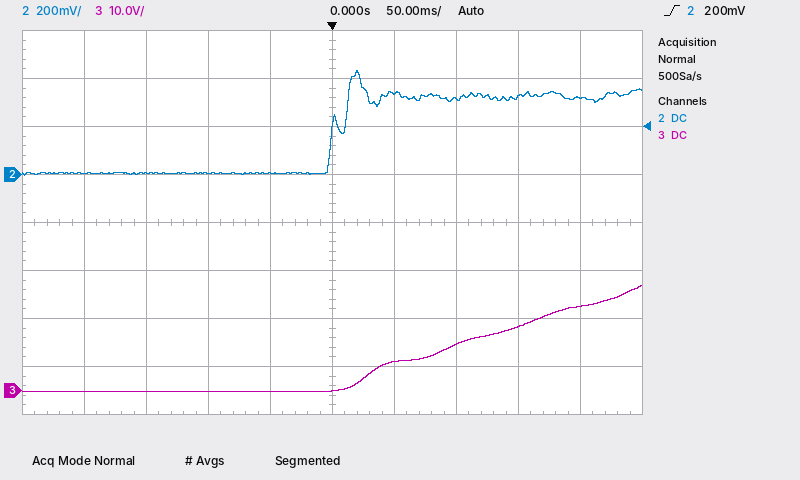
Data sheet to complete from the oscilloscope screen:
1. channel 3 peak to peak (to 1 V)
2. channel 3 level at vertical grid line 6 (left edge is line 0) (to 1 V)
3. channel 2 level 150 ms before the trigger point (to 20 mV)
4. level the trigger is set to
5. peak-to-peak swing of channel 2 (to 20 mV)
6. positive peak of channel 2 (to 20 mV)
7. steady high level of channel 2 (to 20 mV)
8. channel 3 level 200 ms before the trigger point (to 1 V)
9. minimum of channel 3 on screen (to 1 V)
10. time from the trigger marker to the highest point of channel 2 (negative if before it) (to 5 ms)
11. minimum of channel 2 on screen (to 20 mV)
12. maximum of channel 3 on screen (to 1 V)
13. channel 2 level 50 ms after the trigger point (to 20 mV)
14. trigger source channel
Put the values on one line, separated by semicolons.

22 V; 6 V; 0 mV; 200 mV; 440 mV; 440 mV; 320 mV; 0 V; 0 V; +20 ms; 0 mV; 22 V; 340 mV; channel 2
